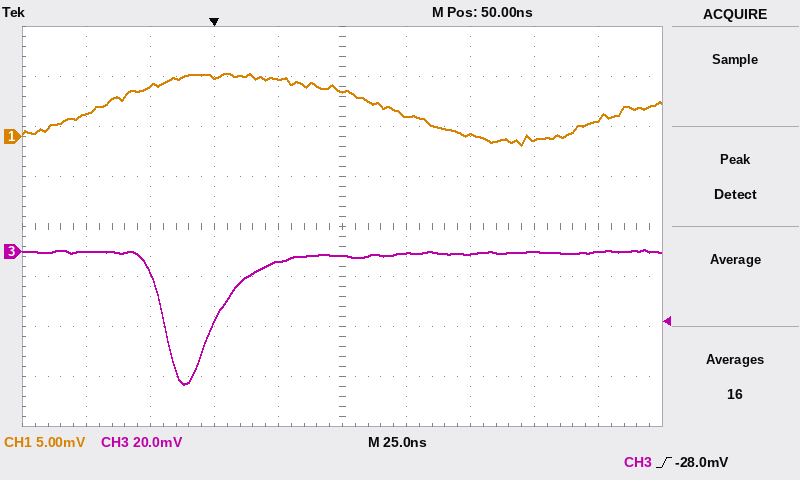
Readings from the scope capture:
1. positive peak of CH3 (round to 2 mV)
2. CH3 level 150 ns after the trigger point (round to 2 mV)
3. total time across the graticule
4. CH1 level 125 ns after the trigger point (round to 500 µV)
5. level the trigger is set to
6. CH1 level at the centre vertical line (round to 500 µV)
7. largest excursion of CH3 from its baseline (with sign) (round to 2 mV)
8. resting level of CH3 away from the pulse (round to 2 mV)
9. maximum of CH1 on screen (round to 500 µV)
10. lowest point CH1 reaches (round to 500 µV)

0 mV
0 mV
250 ns
-500 µV
-28.0 mV
4.5 mV
-52 mV
0 mV
6.5 mV
-1.0 mV
